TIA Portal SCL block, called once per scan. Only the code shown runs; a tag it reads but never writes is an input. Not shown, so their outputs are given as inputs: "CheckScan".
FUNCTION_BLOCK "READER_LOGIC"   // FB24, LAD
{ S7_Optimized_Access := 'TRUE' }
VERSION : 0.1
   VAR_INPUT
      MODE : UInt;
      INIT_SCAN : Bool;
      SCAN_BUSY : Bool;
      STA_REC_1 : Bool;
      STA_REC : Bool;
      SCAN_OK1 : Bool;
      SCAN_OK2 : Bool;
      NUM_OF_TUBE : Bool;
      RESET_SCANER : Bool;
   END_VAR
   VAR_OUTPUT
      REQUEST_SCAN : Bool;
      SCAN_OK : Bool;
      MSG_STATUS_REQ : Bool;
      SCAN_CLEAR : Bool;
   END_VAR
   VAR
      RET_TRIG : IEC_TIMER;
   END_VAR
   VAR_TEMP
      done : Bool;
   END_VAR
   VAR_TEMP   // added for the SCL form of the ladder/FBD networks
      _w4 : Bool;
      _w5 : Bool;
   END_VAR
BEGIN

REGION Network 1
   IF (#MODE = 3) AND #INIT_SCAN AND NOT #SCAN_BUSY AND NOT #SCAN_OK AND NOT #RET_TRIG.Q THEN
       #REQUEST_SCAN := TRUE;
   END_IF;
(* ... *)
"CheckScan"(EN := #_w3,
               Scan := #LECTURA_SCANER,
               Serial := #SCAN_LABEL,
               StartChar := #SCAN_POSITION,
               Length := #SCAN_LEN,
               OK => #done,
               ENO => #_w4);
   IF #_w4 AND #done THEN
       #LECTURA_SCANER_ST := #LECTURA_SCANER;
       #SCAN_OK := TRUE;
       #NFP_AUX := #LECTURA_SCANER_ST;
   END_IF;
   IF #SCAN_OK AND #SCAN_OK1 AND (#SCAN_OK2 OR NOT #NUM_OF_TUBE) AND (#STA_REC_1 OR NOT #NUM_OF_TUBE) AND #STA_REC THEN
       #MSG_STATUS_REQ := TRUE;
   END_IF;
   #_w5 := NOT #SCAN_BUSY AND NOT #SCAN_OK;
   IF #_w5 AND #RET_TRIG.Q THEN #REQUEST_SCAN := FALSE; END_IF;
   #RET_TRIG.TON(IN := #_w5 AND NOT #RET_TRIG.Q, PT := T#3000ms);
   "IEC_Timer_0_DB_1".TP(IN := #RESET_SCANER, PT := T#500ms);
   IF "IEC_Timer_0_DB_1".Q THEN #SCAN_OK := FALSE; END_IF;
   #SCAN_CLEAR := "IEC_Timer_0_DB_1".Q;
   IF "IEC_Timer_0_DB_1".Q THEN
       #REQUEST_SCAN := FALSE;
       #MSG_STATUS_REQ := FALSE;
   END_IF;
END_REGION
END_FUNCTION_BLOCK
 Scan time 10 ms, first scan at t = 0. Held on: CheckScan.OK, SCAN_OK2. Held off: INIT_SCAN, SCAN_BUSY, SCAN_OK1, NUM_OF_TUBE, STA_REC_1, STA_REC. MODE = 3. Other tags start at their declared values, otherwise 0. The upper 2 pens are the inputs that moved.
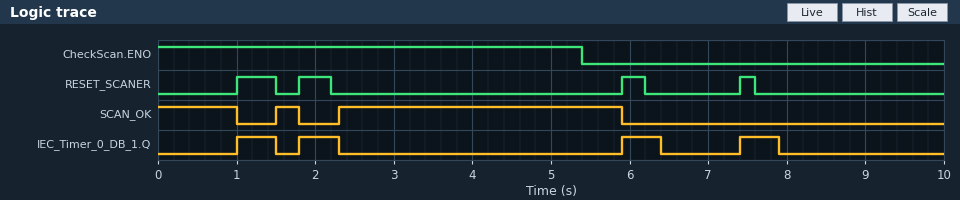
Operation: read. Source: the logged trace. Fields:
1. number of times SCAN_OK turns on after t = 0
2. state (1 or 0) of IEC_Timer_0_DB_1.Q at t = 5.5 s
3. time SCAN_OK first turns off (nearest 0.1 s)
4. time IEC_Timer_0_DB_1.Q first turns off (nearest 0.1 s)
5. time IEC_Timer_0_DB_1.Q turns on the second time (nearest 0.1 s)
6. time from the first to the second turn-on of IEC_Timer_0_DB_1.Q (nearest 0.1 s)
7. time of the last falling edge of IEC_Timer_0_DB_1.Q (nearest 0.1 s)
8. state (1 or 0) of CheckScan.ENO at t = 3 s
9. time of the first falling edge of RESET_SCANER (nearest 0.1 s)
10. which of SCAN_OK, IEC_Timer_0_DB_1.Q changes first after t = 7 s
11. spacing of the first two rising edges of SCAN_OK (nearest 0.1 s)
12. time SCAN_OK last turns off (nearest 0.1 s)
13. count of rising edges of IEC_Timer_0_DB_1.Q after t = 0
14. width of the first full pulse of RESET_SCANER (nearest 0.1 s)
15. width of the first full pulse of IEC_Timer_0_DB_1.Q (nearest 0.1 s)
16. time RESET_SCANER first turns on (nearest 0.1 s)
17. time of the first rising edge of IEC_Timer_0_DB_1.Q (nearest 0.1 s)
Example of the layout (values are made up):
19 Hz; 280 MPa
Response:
2; 0; 1.0 s; 1.5 s; 1.8 s; 0.8 s; 7.9 s; 1; 1.5 s; IEC_Timer_0_DB_1.Q; 0.8 s; 5.9 s; 4; 0.5 s; 0.5 s; 1.0 s; 1.0 s
